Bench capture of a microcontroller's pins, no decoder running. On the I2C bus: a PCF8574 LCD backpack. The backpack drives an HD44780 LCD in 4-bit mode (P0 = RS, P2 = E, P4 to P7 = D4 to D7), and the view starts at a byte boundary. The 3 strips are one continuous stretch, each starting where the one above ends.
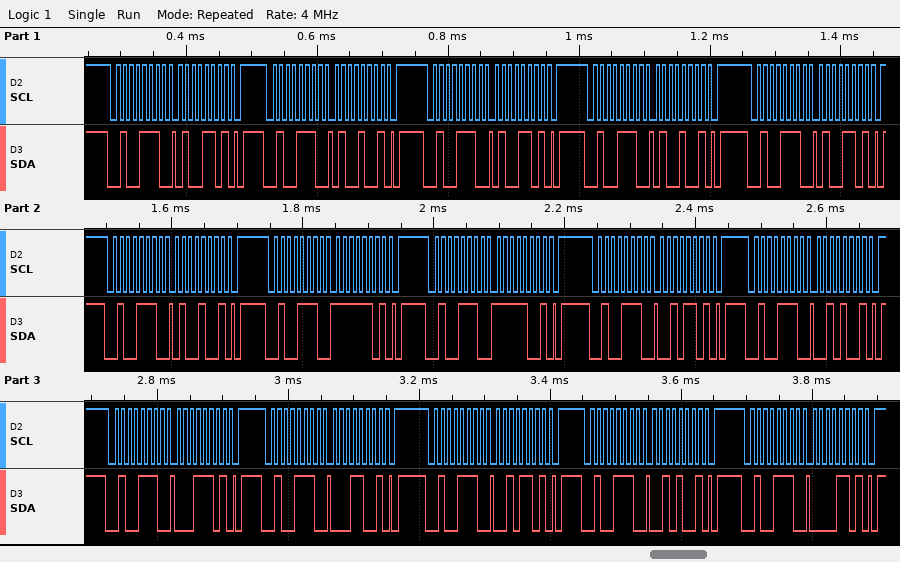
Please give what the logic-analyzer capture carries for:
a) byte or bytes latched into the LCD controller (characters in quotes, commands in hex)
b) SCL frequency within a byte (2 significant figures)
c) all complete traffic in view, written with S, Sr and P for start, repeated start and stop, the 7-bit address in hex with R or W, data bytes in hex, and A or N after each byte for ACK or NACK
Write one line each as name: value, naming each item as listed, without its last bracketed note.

byte or bytes latched into the LCD controller: 'D' 'O' '!'
SCL frequency within a byte: 100 kHz
all complete traffic in view, written with S, Sr and P for start, repeated start and stop, the 7-bit address in hex with R or W, data bytes in hex, and A or N after each byte for ACK or NACK: S 27W A 4D A P S 27W A 49 A P S 27W A 4D A P S 27W A 49 A P S 27W A 4D A P S 27W A 49 A P S 27W A FD A P S 27W A F9 A P S 27W A 2D A P S 27W A 29 A P S 27W A 1D A P S 27W A 19 A P S 27W A 2D A P S 27W A 29 A P S 27W A 0D A P
